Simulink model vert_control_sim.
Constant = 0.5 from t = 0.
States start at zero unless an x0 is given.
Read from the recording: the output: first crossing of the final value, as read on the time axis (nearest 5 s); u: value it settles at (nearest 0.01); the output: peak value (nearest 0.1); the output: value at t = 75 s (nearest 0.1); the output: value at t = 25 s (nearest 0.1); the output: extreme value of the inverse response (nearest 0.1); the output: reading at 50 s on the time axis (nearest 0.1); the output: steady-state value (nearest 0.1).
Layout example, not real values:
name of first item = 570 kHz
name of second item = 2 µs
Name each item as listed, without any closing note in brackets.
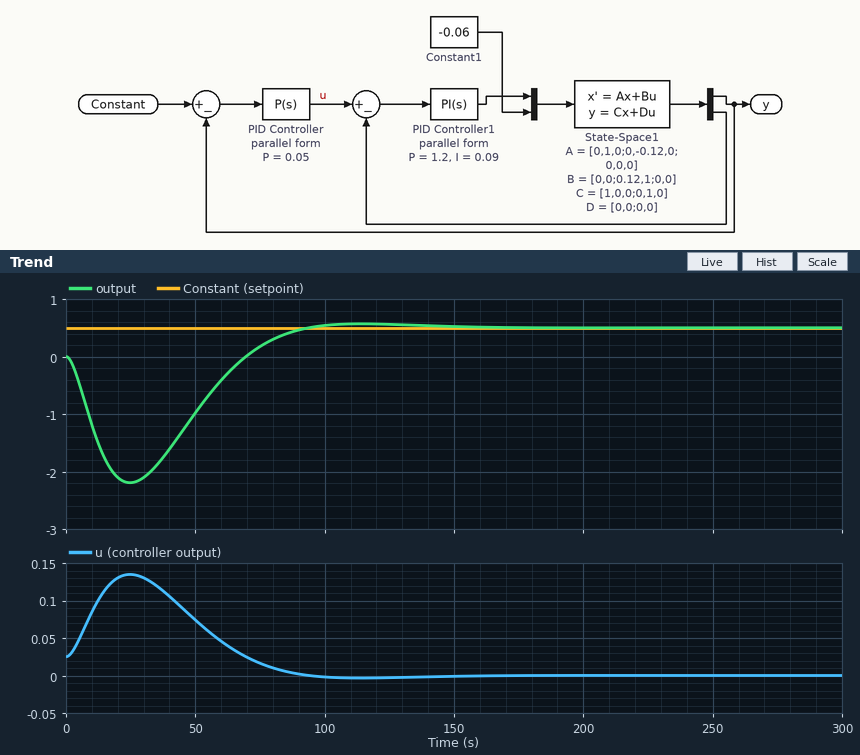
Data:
the output: first crossing of the final value, as read on the time axis = 95 s
u: value it settles at = 0.00
the output: peak value = 0.6
the output: value at t = 75 s = 0.2
the output: value at t = 25 s = -2.2
the output: extreme value of the inverse response = -2.2
the output: reading at 50 s on the time axis = -1.0
the output: steady-state value = 0.5
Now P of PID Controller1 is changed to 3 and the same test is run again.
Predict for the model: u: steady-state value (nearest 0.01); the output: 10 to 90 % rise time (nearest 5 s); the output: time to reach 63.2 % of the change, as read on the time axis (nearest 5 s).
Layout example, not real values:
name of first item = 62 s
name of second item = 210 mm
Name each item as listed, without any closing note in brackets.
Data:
u: steady-state value = 0.00
the output: 10 to 90 % rise time = 60 s
the output: time to reach 63.2 % of the change, as read on the time axis = 120 s
